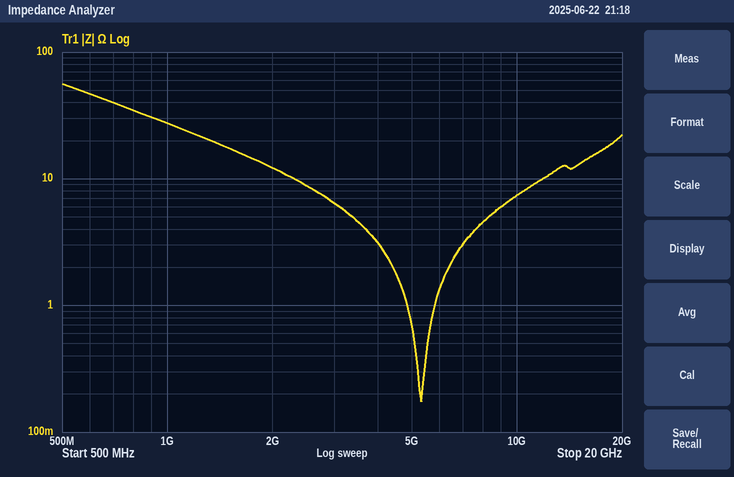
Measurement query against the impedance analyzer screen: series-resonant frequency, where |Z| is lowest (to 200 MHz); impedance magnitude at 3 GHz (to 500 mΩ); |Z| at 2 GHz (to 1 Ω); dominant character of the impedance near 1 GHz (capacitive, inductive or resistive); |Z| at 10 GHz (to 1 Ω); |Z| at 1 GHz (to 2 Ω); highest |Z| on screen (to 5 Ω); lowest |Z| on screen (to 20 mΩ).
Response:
5.4 GHz
6.5 Ω
12 Ω
capacitive
7 Ω
28 Ω
55 Ω
180 mΩ
